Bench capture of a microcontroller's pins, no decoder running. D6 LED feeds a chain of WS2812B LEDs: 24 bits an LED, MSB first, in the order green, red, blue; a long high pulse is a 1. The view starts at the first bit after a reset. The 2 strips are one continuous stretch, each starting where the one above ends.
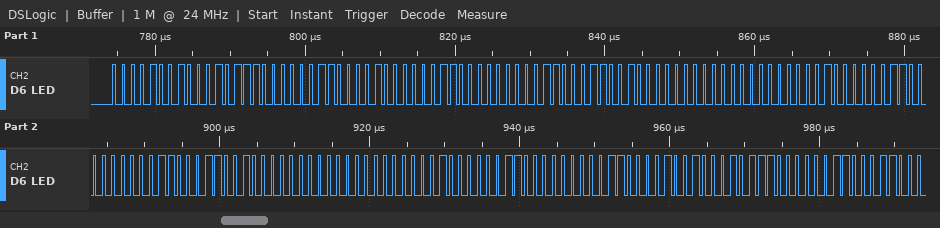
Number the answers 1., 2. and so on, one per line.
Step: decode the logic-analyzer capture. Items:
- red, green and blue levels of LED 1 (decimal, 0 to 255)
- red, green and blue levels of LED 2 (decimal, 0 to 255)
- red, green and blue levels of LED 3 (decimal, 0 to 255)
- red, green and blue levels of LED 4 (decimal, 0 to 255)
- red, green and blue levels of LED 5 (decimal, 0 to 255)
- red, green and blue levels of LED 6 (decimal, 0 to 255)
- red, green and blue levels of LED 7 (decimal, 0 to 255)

1. 23, 9, 3
2. 24, 8, 3
3. 0, 25, 0
4. 24, 8, 3
5. 0, 25, 0
6. 24, 8, 3
7. 23, 9, 3
